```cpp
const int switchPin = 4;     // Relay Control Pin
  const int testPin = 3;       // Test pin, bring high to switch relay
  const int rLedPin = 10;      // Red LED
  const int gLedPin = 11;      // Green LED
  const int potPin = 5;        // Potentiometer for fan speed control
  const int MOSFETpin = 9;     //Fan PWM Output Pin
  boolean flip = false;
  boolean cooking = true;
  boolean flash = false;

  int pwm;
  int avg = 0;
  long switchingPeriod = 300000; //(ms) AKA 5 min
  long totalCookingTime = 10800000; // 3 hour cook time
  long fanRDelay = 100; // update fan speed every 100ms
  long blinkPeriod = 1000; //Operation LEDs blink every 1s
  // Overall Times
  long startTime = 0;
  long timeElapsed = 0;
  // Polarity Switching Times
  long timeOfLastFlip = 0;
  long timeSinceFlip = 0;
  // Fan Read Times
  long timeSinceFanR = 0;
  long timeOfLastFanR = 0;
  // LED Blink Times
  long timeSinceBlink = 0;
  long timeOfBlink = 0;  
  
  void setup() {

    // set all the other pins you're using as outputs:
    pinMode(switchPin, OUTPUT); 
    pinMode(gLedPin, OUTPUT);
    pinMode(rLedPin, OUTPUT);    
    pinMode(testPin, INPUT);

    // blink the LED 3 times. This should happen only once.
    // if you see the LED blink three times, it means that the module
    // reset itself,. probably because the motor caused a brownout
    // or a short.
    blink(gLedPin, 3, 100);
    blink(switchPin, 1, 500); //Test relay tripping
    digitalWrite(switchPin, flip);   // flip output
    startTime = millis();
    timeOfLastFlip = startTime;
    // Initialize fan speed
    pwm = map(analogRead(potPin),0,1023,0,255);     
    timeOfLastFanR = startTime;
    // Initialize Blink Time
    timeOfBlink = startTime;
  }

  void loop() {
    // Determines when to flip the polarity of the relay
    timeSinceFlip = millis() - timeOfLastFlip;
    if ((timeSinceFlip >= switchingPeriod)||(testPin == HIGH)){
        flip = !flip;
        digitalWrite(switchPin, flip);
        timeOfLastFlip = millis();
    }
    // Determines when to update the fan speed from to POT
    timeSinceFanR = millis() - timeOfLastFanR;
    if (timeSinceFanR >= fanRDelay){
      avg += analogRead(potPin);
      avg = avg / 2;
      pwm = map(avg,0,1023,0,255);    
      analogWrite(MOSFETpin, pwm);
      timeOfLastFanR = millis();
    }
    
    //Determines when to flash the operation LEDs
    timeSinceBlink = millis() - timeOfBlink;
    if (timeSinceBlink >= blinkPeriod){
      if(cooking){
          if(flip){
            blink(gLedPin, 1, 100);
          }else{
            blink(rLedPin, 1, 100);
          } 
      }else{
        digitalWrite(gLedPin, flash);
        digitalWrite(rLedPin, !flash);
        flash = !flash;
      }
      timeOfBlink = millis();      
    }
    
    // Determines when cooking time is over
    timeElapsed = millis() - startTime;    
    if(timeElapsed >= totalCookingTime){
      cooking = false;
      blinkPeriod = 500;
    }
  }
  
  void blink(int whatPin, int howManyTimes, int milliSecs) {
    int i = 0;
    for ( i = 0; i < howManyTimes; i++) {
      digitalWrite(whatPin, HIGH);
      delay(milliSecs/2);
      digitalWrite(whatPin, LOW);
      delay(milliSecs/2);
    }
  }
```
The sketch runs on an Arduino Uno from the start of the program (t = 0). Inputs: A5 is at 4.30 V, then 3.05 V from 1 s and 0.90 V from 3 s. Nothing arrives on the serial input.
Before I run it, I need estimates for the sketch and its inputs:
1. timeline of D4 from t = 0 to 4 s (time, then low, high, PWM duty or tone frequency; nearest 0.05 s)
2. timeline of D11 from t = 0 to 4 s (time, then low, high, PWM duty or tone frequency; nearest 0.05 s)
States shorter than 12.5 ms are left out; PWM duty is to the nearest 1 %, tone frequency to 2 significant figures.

0 s low; 0.3 s high; 0.55 s low
0 s high; 0.05 s low; 0.1 s high; 0.15 s low; 0.2 s high; 0.25 s low
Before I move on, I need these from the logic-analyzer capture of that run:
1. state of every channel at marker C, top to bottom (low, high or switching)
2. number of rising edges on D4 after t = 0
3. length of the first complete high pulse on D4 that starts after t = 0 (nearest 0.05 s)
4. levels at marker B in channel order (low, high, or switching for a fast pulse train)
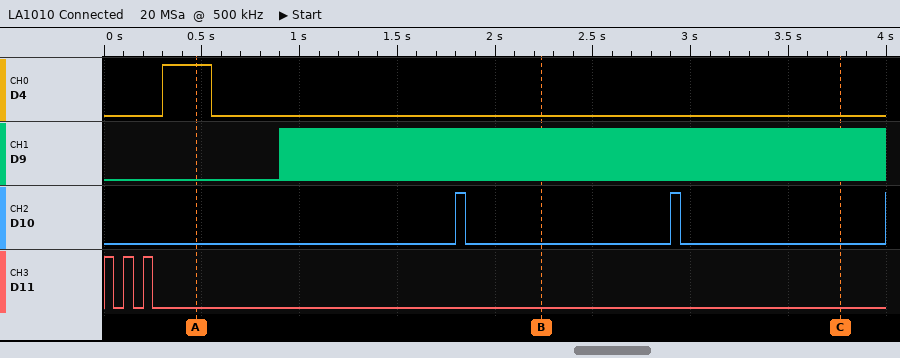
D4 low, D9 switching, D10 low, D11 low
1
0.25 s
D4 low, D9 switching, D10 low, D11 low
